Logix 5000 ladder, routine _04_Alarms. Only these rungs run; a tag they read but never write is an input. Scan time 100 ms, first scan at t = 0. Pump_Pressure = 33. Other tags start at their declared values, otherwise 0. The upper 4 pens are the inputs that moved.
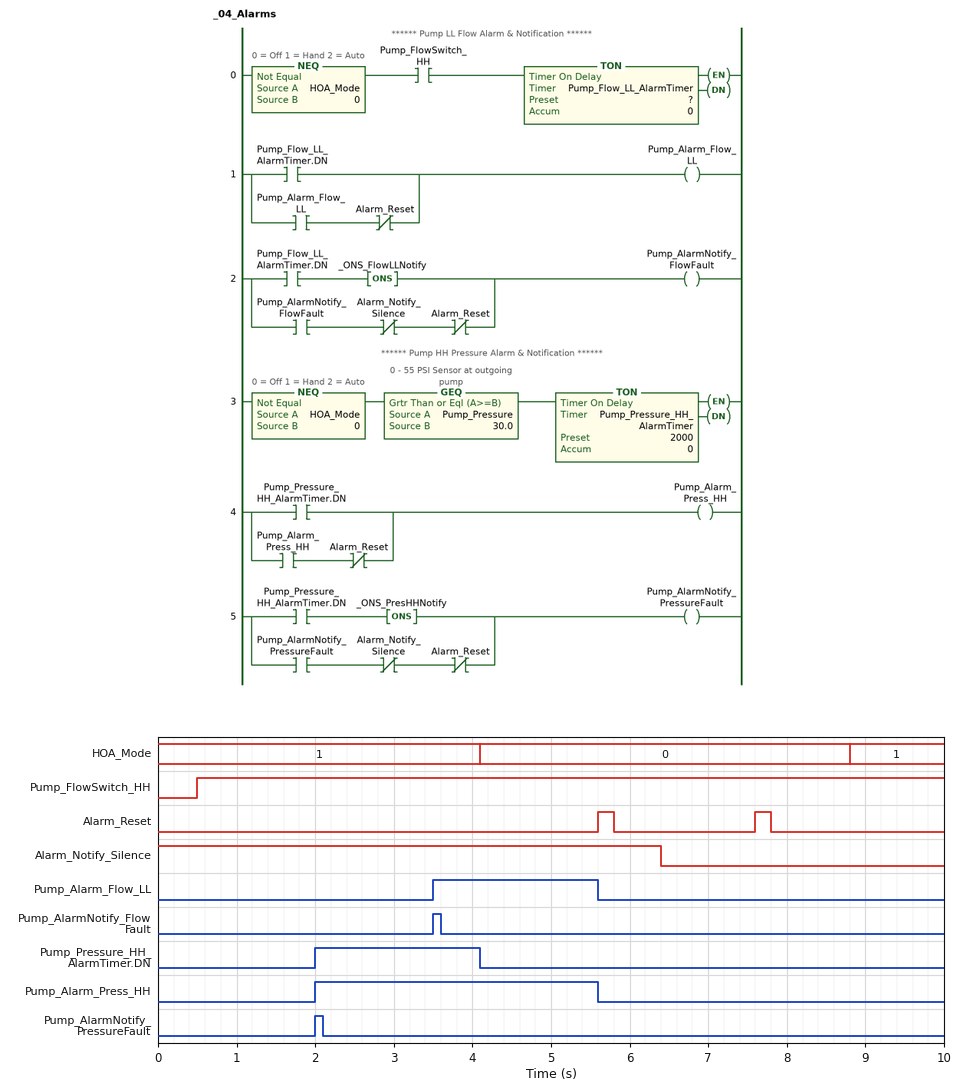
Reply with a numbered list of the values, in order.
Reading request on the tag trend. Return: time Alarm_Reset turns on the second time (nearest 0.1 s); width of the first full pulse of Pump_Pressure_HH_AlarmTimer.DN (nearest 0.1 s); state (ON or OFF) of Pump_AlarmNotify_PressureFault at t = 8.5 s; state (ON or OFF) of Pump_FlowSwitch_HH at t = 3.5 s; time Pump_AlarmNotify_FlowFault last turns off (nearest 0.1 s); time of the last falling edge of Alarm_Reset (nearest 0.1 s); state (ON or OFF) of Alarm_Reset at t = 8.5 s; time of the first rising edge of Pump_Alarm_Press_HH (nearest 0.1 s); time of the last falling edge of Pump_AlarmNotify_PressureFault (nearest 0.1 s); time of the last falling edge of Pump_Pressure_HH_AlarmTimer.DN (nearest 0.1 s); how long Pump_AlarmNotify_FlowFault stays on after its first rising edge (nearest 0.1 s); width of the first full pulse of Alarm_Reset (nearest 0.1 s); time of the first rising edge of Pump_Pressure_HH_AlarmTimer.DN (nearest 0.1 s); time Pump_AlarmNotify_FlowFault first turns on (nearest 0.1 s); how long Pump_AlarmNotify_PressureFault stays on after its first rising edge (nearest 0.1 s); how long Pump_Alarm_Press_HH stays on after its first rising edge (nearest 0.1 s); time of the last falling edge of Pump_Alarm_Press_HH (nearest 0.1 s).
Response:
1. 7.6 s
2. 2.1 s
3. OFF
4. ON
5. 3.6 s
6. 7.8 s
7. OFF
8. 2.0 s
9. 2.1 s
10. 4.1 s
11. 0.1 s
12. 0.2 s
13. 2.0 s
14. 3.5 s
15. 0.1 s
16. 3.6 s
17. 5.6 s
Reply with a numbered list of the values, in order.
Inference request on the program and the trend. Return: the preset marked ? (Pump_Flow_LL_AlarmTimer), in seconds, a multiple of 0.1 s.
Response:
1. 3.0 s
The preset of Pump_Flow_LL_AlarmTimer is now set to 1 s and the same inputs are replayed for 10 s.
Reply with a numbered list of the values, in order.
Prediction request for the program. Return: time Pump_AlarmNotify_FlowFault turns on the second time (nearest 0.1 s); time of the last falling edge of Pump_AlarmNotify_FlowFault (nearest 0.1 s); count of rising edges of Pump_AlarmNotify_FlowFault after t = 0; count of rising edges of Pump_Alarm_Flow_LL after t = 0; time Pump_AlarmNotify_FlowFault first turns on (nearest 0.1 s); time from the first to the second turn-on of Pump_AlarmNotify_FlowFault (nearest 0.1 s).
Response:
1. 9.8 s
2. 1.6 s
3. 2
4. 2
5. 1.5 s
6. 8.3 s
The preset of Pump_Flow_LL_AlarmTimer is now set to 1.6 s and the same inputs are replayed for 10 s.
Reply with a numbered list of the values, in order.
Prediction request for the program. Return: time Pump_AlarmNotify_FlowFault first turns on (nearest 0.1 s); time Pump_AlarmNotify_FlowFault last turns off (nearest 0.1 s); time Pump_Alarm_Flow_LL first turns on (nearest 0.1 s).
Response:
1. 2.1 s
2. 2.2 s
3. 2.1 s
